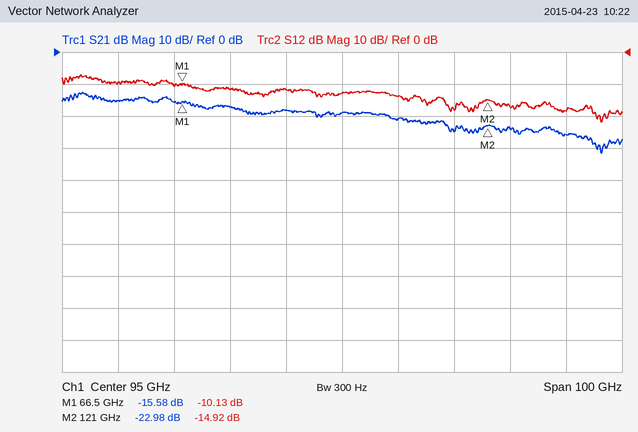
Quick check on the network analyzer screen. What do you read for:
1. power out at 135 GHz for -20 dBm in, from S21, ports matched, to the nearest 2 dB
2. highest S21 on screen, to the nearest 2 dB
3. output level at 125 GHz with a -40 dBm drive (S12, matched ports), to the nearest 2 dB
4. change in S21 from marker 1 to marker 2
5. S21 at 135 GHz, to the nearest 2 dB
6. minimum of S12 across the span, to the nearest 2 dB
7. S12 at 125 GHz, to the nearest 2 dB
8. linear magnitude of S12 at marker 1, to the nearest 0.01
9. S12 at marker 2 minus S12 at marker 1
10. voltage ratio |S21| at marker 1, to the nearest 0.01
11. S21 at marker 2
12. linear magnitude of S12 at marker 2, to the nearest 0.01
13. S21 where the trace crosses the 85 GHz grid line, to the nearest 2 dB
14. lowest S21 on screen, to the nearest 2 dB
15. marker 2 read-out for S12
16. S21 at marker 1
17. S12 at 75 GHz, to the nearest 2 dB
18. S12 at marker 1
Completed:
-46 dBm
-12 dB
-58 dBm
-7.40 dB
-26 dB
-22 dB
-18 dB
0.31
-4.79 dB
0.17
-22.98 dB
0.18
-18 dB
-32 dB
-14.92 dB
-15.58 dB
-12 dB
-10.13 dB
